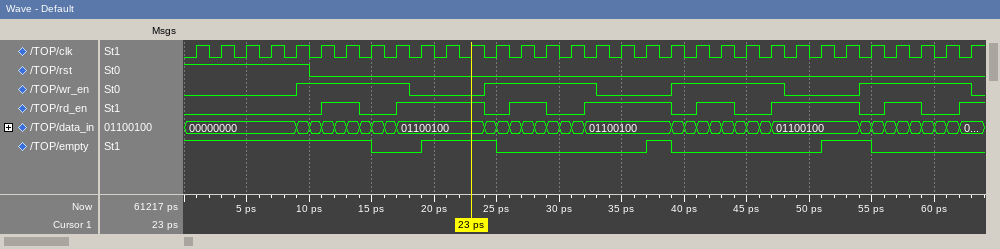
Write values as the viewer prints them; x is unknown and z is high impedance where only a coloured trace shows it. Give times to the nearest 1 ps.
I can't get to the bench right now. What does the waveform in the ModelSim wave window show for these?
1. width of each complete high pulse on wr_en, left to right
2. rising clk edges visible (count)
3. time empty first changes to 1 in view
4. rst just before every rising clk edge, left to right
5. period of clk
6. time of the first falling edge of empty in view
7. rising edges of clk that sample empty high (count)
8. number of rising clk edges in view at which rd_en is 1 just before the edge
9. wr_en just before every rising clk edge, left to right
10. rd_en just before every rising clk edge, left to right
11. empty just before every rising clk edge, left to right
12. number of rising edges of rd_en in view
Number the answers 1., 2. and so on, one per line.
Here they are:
1. 9 ps, 9 ps, 9 ps, 9 ps
2. 32
3. 19 ps
4. 1 1 1 1 1 0 0 0 0 0 0 0 0 0 0 0 0 0 0 0 0 0 0 0 0 0 0 0 0 0 0 0
5. 2 ps
6. 15 ps
7. 14
8. 17
9. 0 0 0 0 0 1 1 1 1 0 0 0 1 1 1 1 1 0 0 0 1 1 1 1 0 0 0 1 1 1 1 1
10. 0 0 0 0 0 0 1 0 0 1 1 1 0 1 1 0 1 1 1 1 0 1 0 0 1 1 1 0 1 1 0 1
11. 1 1 1 1 1 1 1 1 0 0 1 1 1 0 0 0 0 0 0 1 0 0 0 0 0 0 1 1 0 0 0 0
12. 8
